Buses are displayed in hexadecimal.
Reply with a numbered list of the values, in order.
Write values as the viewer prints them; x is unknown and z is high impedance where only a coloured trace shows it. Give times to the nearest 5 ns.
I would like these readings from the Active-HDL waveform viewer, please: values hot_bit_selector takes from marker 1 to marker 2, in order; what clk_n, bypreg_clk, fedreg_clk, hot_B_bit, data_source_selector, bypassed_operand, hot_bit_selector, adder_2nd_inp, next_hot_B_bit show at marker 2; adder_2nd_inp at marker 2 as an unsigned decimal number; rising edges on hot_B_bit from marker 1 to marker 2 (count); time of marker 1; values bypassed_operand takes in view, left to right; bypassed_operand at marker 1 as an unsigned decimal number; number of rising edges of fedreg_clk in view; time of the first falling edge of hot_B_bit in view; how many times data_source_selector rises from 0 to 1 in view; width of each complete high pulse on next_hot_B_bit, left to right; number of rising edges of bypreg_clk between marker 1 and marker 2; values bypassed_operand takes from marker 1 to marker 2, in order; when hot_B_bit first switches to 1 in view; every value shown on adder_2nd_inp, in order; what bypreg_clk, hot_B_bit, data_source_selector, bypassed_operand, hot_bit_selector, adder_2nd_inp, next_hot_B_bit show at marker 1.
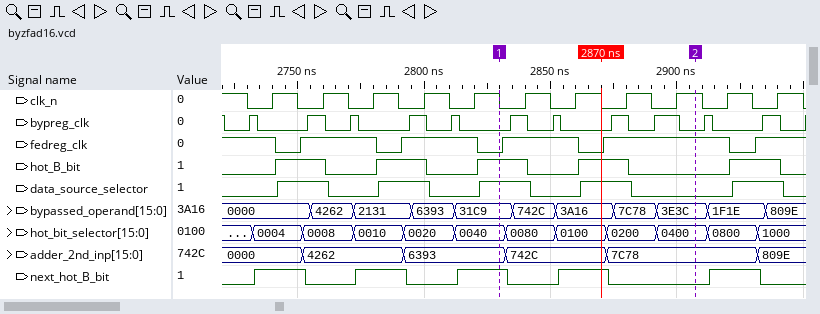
1. 0040, 0080, 0100, 0200, 0400
2. clk_n=1, bypreg_clk=0, fedreg_clk=1, hot_B_bit=0, data_source_selector=0, bypassed_operand=3E3C, hot_bit_selector=0400, adder_2nd_inp=7C78, next_hot_B_bit=0
3. 31864
4. 1
5. 2830 ns
6. 0000, 4262, 2131, 6393, 31C9, 742C, 3A16, 7C78, 3E3C, 1F1E, 809E
7. 12745
8. 5
9. 2760 ns
10. 5
11. 20 ns, 20 ns, 20 ns, 20 ns, 20 ns
12. 4
13. 31C9, 742C, 3A16, 7C78, 3E3C
14. 2740 ns
15. 0000, 4262, 6393, 742C, 7C78, 809E
16. bypreg_clk=0, hot_B_bit=1, data_source_selector=1, bypassed_operand=31C9, hot_bit_selector=0040, adder_2nd_inp=6393, next_hot_B_bit=1
